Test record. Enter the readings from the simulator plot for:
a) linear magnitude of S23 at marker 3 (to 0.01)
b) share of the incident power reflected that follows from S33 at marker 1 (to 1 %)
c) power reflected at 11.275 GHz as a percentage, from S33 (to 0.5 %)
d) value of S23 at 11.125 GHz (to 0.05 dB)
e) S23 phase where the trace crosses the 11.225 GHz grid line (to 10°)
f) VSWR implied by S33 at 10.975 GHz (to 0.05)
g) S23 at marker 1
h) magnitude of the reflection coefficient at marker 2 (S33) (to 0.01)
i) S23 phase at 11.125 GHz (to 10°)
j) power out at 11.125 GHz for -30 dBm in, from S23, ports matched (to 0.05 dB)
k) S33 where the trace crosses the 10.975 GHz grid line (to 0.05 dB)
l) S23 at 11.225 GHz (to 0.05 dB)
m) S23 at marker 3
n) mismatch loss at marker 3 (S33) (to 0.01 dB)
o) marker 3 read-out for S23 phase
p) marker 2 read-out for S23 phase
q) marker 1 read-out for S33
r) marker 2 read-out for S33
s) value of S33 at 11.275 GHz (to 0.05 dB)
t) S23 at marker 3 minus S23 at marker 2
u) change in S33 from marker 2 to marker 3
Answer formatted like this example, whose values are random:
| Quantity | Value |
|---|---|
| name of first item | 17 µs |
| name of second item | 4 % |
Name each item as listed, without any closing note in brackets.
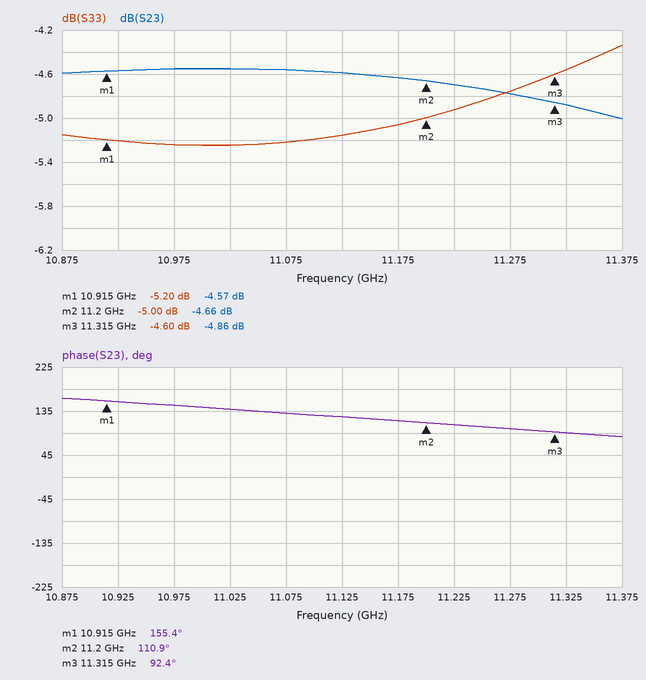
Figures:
| Quantity | Value |
|---|---|
| linear magnitude of S23 at marker 3 | 0.57 |
| share of the incident power reflected that follows from S33 at marker 1 | 30 % |
| power reflected at 11.275 GHz as a percentage, from S33 | 33.5 % |
| value of S23 at 11.125 GHz | -4.60 dB |
| S23 phase where the trace crosses the 11.225 GHz grid line | 110° |
| VSWR implied by S33 at 10.975 GHz | 3.40 |
| S23 at marker 1 | -4.57 dB |
| magnitude of the reflection coefficient at marker 2 (S33) | 0.56 |
| S23 phase at 11.125 GHz | 120° |
| power out at 11.125 GHz for -30 dBm in, from S23, ports matched | -34.60 dBm |
| S33 where the trace crosses the 10.975 GHz grid line | -5.25 dB |
| S23 at 11.225 GHz | -4.70 dB |
| S23 at marker 3 | -4.86 dB |
| mismatch loss at marker 3 (S33) | 1.85 dB |
| marker 3 read-out for S23 phase | 92.4° |
| marker 2 read-out for S23 phase | 110.9° |
| marker 1 read-out for S33 | -5.20 dB |
| marker 2 read-out for S33 | -5.00 dB |
| value of S33 at 11.275 GHz | -4.75 dB |
| S23 at marker 3 minus S23 at marker 2 | -0.20 dB |
| change in S33 from marker 2 to marker 3 | 0.40 dB |
